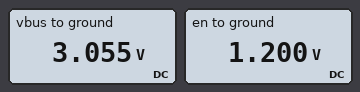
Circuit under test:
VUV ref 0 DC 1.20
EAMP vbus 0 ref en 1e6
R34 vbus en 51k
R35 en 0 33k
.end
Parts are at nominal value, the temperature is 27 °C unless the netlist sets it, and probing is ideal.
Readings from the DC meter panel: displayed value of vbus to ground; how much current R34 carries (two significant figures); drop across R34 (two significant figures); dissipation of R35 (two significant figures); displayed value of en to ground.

3.055 V
36 µA
1.9 V
44 µW
1.200 V
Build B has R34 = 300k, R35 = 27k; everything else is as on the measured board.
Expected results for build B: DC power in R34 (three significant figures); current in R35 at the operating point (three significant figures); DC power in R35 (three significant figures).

593 µW
44.4 µA
53.3 µW
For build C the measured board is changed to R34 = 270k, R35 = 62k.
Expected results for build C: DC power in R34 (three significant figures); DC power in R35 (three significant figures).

101 µW
23.2 µW
